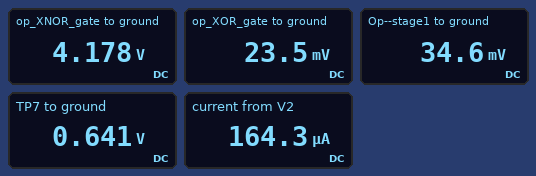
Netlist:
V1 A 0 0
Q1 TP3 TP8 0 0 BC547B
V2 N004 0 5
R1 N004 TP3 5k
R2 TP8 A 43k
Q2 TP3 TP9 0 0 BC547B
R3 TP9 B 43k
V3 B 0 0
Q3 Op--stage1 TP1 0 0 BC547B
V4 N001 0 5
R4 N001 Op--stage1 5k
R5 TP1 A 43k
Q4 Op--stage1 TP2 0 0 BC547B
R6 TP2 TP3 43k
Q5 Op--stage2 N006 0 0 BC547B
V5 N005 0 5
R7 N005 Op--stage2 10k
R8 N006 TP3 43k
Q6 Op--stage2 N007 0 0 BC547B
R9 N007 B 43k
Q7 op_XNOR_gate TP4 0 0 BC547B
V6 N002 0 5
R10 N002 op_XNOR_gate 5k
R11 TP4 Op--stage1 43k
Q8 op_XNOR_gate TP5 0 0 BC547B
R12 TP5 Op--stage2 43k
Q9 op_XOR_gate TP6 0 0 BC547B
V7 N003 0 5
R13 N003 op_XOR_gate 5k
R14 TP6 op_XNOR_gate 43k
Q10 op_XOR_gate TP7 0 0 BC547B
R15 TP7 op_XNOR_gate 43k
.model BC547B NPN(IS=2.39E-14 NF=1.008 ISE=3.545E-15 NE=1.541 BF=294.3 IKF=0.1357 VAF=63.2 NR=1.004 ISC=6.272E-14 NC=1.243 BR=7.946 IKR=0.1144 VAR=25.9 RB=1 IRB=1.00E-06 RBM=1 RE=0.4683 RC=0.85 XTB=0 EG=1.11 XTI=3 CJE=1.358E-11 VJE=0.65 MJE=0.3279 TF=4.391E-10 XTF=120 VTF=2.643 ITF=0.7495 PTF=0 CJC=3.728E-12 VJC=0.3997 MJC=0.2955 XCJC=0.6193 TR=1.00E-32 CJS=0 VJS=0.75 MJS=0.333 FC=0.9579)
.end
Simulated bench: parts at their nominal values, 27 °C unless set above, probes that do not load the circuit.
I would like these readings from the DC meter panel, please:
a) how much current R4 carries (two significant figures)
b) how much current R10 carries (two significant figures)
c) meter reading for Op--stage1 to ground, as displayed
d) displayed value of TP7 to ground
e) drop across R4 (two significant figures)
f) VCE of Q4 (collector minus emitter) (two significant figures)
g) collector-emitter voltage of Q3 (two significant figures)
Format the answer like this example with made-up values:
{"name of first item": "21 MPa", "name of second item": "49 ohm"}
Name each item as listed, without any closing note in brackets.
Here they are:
{"how much current R4 carries": "990 µA", "how much current R10 carries": "160 µA", "meter reading for Op--stage1 to ground, as displayed": "34.6 mV", "displayed value of TP7 to ground": "0.641 V", "drop across R4": "5.0 V", "VCE of Q4 (collector minus emitter)": "35 mV", "collector-emitter voltage of Q3": "35 mV"}
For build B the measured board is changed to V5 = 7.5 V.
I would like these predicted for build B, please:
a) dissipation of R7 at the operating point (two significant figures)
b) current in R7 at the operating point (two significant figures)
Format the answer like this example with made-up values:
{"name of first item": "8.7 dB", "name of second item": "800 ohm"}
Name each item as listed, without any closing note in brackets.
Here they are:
{"dissipation of R7 at the operating point": "5.6 mW", "current in R7 at the operating point": "750 µA"}
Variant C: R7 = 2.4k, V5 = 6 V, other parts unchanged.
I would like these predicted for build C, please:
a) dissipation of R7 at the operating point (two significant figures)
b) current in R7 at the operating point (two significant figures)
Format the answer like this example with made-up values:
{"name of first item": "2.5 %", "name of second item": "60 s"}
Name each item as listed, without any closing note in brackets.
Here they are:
{"dissipation of R7 at the operating point": "15 mW", "current in R7 at the operating point": "2.5 mA"}
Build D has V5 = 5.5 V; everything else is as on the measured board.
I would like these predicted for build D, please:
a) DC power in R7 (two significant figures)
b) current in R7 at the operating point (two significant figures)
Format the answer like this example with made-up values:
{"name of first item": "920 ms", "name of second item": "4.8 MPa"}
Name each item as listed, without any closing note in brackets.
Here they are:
{"DC power in R7": "3.0 mW", "current in R7 at the operating point": "550 µA"}
